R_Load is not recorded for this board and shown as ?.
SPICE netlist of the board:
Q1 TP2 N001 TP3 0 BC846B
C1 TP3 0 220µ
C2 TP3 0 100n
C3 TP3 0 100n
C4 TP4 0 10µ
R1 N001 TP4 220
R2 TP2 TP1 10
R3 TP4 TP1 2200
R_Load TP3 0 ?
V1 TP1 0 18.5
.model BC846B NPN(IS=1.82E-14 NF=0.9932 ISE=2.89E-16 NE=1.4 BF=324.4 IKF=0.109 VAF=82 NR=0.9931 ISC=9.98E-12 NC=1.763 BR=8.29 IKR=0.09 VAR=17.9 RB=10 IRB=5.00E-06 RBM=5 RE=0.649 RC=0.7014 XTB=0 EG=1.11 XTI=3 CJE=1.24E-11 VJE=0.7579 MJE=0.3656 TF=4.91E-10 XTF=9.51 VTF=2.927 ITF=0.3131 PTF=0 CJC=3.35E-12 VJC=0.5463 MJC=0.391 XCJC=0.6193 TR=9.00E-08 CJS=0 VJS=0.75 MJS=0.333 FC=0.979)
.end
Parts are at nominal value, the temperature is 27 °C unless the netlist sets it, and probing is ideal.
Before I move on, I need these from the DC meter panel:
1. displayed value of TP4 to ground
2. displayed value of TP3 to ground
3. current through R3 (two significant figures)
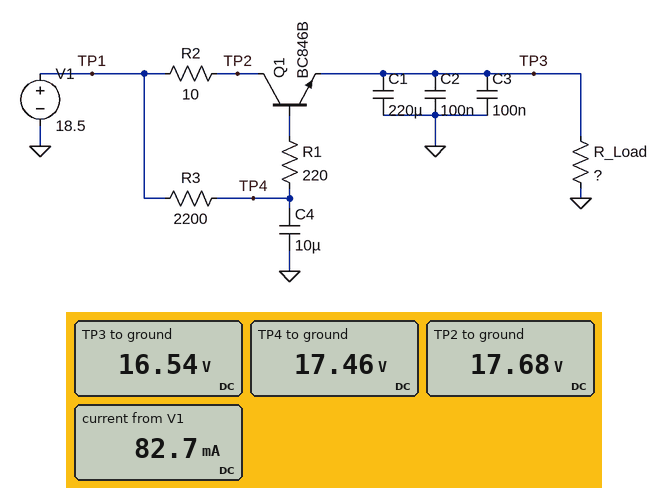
17.46 V
16.54 V
470 µA
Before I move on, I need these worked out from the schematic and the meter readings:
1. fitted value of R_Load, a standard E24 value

200 Ω
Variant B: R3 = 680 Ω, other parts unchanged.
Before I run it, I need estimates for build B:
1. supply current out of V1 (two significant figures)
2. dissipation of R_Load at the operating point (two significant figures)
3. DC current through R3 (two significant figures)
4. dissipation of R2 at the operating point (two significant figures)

86 mA
1.5 W
510 µA
73 mW
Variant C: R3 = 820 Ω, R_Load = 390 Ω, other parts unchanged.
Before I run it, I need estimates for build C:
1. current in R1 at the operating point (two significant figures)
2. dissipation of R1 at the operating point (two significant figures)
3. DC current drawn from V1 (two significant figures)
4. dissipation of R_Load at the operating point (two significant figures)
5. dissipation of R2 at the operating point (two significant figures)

210 µA
9.4 µW
45 mA
790 mW
20 mW
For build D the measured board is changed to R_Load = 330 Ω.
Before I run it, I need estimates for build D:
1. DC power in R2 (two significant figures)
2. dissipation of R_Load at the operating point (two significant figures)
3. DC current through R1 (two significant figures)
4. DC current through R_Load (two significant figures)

27 mW
890 mW
250 µA
52 mA
